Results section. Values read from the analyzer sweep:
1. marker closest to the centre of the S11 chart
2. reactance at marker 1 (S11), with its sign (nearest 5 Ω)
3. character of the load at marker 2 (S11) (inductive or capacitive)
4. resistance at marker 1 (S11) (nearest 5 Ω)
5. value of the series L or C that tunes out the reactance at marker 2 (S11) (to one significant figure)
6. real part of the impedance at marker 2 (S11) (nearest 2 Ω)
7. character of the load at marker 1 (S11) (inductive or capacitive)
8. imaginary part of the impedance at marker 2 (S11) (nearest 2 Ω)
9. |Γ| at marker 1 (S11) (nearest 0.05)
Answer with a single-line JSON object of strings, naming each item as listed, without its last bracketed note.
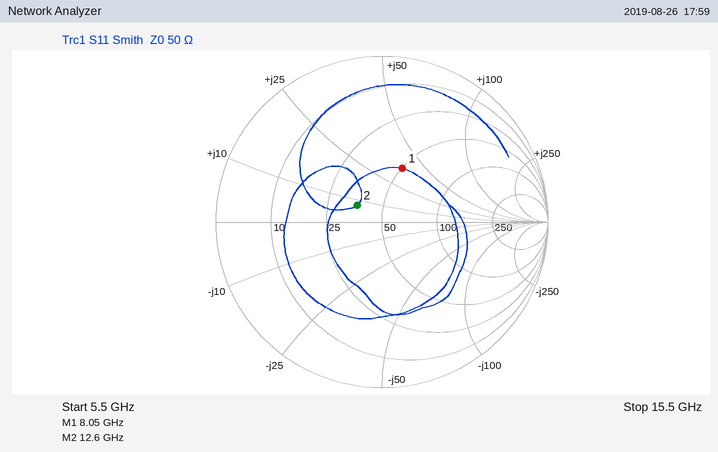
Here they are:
{"marker closest to the centre of the S11 chart": "marker 2", "reactance at marker 1 (S11), with its sign": "+35 Ω", "character of the load at marker 2 (S11)": "inductive", "resistance at marker 1 (S11)": "50 Ω", "value of the series L or C that tunes out the reactance at marker 2 (S11)": "2 pF", "real part of the impedance at marker 2 (S11)": "36 Ω", "character of the load at marker 1 (S11)": "inductive", "imaginary part of the impedance at marker 2 (S11)": "+8 Ω", "|Γ| at marker 1 (S11)": "0.35"}
